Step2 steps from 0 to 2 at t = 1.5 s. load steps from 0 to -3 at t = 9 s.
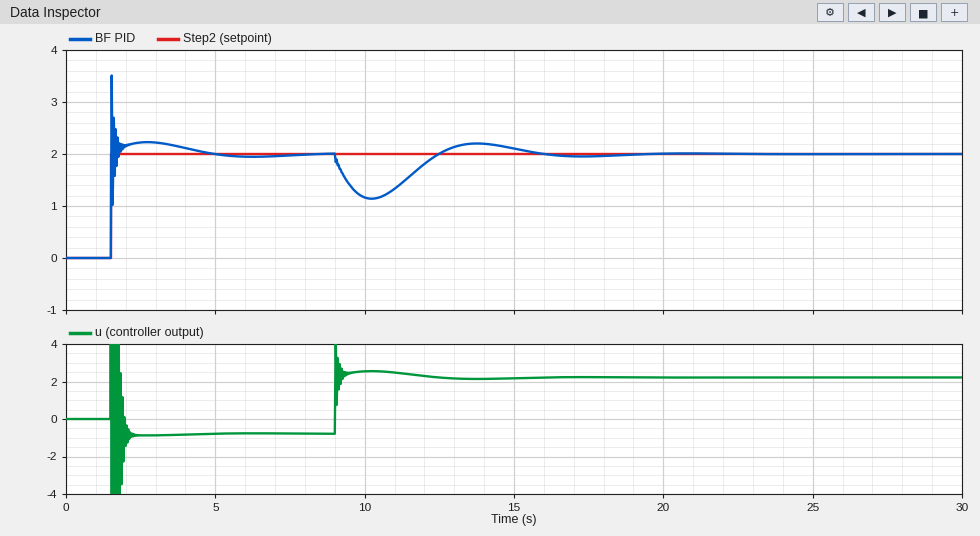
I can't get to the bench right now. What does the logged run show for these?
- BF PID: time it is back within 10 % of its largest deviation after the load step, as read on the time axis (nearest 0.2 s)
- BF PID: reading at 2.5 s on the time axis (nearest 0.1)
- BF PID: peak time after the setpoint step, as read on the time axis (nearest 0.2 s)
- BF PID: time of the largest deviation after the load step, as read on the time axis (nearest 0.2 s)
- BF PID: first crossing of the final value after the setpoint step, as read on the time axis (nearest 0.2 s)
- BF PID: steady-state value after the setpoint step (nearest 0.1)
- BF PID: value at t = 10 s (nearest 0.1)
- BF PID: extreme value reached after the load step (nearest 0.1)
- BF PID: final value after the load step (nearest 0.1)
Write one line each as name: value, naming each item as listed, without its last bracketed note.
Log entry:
BF PID: time it is back within 10 % of its largest deviation after the load step, as read on the time axis: 15.2 s
BF PID: reading at 2.5 s on the time axis: 2.2
BF PID: peak time after the setpoint step, as read on the time axis: 1.6 s
BF PID: time of the largest deviation after the load step, as read on the time axis: 10.2 s
BF PID: first crossing of the final value after the setpoint step, as read on the time axis: 1.6 s
BF PID: steady-state value after the setpoint step: 2.0
BF PID: value at t = 10 s: 1.2
BF PID: extreme value reached after the load step: 1.1
BF PID: final value after the load step: 2.0
